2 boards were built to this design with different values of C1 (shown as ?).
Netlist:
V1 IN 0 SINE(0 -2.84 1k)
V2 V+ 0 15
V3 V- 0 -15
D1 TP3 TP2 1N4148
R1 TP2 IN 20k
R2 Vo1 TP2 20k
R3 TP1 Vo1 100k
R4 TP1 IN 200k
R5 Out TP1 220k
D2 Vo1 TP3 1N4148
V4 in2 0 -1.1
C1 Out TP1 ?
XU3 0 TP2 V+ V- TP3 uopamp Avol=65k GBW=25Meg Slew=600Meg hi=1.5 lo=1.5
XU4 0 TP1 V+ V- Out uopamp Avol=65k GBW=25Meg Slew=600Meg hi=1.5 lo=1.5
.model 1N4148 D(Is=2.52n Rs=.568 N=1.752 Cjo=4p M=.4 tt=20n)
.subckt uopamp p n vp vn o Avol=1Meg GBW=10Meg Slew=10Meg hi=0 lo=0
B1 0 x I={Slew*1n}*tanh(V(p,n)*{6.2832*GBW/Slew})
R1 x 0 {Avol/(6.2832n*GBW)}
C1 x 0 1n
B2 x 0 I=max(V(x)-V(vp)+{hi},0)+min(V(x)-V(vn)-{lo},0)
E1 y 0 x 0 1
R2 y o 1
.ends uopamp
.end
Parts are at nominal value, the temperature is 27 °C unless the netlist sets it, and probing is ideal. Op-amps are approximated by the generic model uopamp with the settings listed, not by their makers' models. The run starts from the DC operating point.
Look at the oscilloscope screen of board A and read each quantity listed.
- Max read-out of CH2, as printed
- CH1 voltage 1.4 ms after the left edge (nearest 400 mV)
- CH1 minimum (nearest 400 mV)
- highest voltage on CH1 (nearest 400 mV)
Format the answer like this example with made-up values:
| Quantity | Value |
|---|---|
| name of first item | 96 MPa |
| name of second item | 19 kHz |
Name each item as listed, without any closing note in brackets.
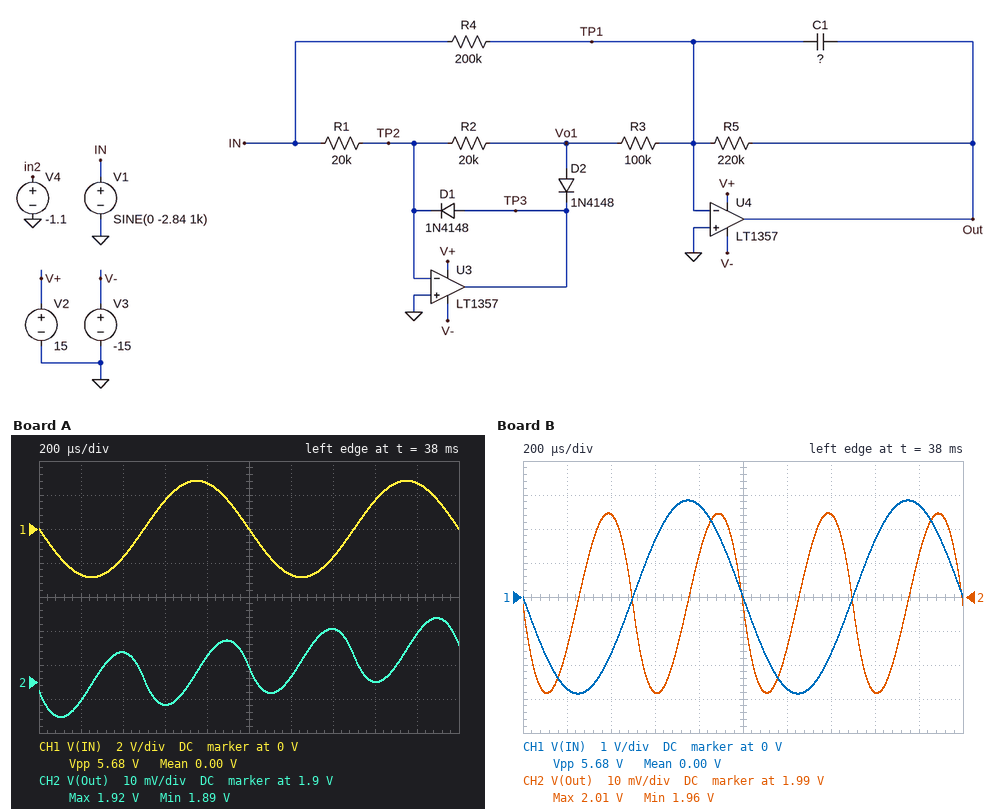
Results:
| Quantity | Value |
|---|---|
| Max read-out of CH2, as printed | 1.92 V |
| CH1 voltage 1.4 ms after the left edge | -1.6 V |
| CH1 minimum | -2.8 V |
| highest voltage on CH1 | 2.8 V |
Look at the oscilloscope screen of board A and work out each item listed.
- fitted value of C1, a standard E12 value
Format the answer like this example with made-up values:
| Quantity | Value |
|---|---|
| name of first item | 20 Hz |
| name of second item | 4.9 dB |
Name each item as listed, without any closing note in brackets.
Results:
| Quantity | Value |
|---|---|
| fitted value of C1, a standard E12 value | 56 nF |
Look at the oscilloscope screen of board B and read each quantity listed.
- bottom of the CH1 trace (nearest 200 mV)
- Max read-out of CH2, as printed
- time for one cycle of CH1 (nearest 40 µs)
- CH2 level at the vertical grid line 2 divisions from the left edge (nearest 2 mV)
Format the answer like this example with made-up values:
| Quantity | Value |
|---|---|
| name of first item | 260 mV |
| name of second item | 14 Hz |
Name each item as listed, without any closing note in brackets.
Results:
| Quantity | Value |
|---|---|
| bottom of the CH1 trace | -2.8 V |
| Max read-out of CH2, as printed | 2.01 V |
| time for one cycle of CH1 | 1.00 ms |
| CH2 level at the vertical grid line 2 divisions from the left edge | 2.014 V |
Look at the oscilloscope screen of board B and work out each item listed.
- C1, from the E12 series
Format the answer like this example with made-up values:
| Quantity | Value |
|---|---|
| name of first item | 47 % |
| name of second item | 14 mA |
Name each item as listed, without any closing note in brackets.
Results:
| Quantity | Value |
|---|---|
| C1, from the E12 series | 18 nF |
